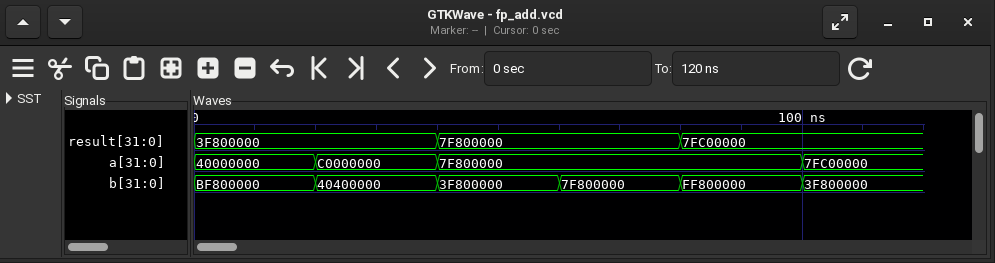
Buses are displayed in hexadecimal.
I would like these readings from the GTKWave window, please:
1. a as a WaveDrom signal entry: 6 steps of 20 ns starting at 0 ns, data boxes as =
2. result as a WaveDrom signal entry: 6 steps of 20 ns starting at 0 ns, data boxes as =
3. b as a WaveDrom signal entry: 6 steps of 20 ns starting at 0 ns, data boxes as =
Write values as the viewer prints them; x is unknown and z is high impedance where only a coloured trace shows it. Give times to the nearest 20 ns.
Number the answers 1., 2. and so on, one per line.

1. {name: 'a', wave: '===..=', data: '40000000 C0000000 7F800000 7FC00000'}
2. {name: 'result', wave: '=.=.=.', data: '3F800000 7F800000 7FC00000'}
3. {name: 'b', wave: '======', data: 'BF800000 40400000 3F800000 7F800000 FF800000 3F800000'}
